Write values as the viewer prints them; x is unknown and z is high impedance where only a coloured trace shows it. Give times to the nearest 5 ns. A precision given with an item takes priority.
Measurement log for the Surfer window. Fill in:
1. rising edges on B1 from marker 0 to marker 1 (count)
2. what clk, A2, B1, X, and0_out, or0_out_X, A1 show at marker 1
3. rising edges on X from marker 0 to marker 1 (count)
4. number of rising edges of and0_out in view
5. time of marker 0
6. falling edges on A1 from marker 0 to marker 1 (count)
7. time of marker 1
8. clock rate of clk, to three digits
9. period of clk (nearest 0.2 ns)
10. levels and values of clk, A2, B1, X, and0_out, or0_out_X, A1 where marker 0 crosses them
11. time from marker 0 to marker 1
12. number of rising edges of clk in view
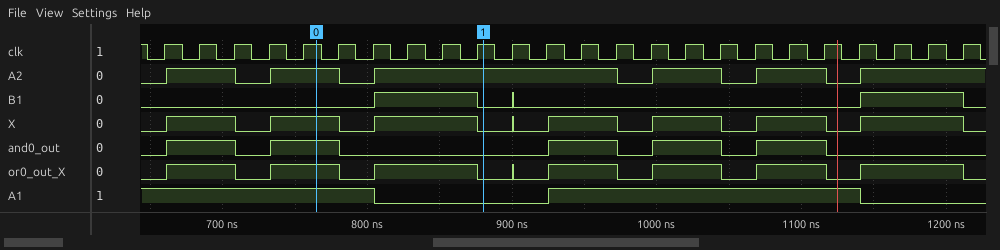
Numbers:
1
clk=1, A2=1, B1=0, X=0, and0_out=0, or0_out_X=0, A1=0
1
5
765 ns
1
880 ns
41.7 MHz
24 ns
clk=1, A2=1, B1=0, X=1, and0_out=1, or0_out_X=1, A1=1
115 ns
24
